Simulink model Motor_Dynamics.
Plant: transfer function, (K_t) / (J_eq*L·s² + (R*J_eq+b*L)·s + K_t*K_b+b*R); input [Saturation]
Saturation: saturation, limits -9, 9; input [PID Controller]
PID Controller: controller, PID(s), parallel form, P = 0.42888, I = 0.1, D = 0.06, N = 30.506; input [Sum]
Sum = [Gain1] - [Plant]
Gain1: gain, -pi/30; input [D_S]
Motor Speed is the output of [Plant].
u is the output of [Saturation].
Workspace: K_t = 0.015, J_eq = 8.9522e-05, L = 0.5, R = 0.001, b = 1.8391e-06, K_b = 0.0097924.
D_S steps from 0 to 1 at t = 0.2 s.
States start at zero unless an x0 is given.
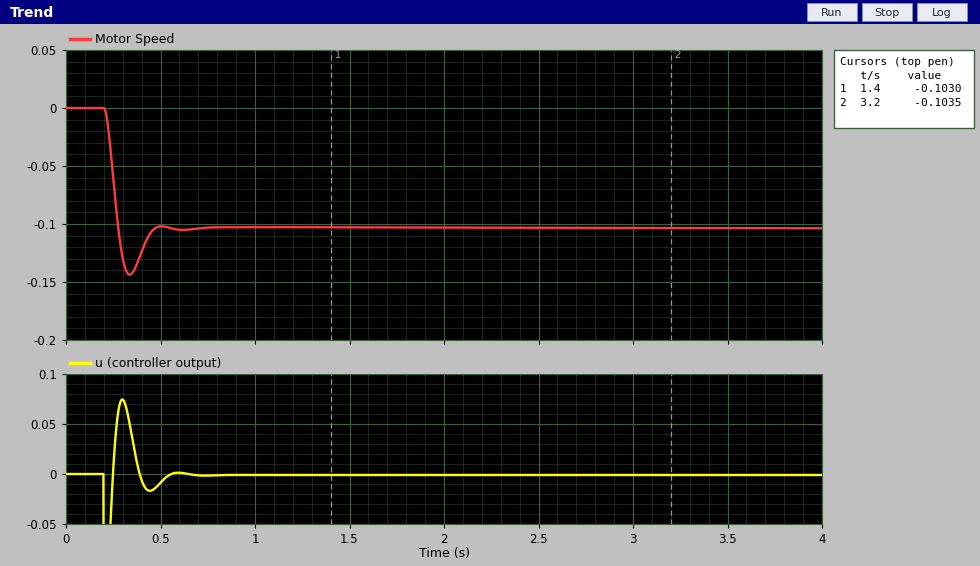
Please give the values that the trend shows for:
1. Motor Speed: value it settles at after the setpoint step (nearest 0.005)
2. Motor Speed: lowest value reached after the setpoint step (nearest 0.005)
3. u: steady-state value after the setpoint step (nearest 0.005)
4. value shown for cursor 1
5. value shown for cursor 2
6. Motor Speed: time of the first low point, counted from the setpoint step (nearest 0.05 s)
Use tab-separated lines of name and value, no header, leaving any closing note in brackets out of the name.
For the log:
Motor Speed: value it settles at after the setpoint step	-0.105
Motor Speed: lowest value reached after the setpoint step	-0.145
u: steady-state value after the setpoint step	0.000
value shown for cursor 1	-0.1030
value shown for cursor 2	-0.1035
Motor Speed: time of the first low point, counted from the setpoint step	0.15 s
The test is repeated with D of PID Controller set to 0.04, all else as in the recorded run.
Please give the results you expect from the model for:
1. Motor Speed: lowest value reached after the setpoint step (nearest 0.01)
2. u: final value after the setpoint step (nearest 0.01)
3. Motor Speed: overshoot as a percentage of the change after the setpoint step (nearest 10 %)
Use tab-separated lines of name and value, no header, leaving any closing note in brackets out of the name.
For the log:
Motor Speed: lowest value reached after the setpoint step	-0.15
u: final value after the setpoint step	0.00
Motor Speed: overshoot as a percentage of the change after the setpoint step	40 %
